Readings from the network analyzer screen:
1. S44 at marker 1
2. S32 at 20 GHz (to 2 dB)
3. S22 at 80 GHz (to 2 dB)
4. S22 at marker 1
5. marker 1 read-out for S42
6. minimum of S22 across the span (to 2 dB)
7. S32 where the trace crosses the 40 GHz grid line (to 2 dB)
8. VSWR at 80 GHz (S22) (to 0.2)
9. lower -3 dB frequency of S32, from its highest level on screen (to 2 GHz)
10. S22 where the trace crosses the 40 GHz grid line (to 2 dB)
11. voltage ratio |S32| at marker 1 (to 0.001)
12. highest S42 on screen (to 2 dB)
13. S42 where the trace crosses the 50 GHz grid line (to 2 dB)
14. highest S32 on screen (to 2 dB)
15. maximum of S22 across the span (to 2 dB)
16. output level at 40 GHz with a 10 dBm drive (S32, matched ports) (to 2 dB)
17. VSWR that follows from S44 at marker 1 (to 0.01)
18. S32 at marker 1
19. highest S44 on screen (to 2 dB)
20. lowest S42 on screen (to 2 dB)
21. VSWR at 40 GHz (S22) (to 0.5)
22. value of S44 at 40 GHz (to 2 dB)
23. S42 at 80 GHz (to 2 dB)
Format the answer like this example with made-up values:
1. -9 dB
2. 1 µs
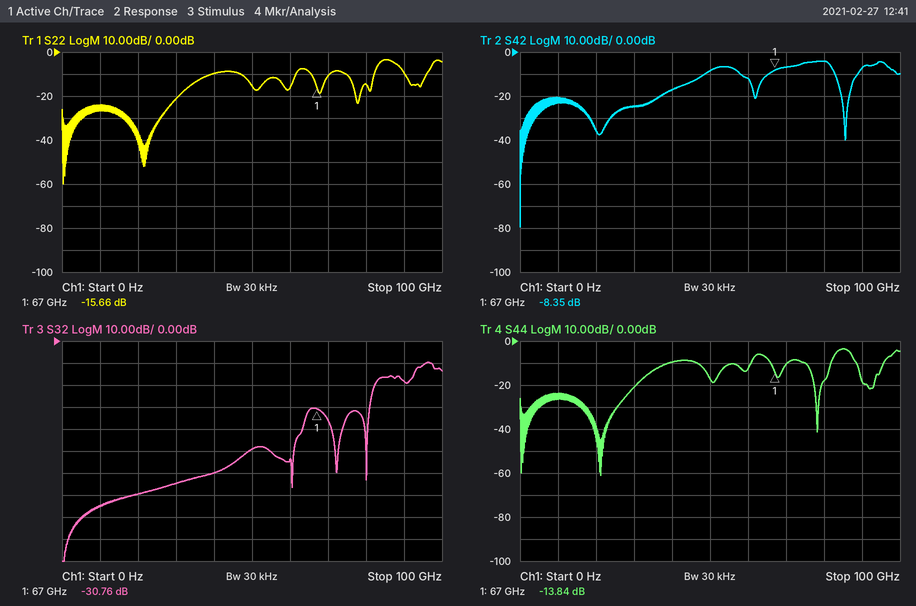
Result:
1. -13.84 dB
2. -70 dB
3. -14 dB
4. -15.66 dB
5. -8.35 dB
6. -60 dB
7. -60 dB
8. 1.4
9. 94 GHz
10. -10 dB
11. 0.029
12. -4 dB
13. -8 dB
14. -10 dB
15. -4 dB
16. -50 dBm
17. 1.51
18. -30.76 dB
19. -4 dB
20. -80 dB
21. 2.0
22. -10 dB
23. -4 dB
